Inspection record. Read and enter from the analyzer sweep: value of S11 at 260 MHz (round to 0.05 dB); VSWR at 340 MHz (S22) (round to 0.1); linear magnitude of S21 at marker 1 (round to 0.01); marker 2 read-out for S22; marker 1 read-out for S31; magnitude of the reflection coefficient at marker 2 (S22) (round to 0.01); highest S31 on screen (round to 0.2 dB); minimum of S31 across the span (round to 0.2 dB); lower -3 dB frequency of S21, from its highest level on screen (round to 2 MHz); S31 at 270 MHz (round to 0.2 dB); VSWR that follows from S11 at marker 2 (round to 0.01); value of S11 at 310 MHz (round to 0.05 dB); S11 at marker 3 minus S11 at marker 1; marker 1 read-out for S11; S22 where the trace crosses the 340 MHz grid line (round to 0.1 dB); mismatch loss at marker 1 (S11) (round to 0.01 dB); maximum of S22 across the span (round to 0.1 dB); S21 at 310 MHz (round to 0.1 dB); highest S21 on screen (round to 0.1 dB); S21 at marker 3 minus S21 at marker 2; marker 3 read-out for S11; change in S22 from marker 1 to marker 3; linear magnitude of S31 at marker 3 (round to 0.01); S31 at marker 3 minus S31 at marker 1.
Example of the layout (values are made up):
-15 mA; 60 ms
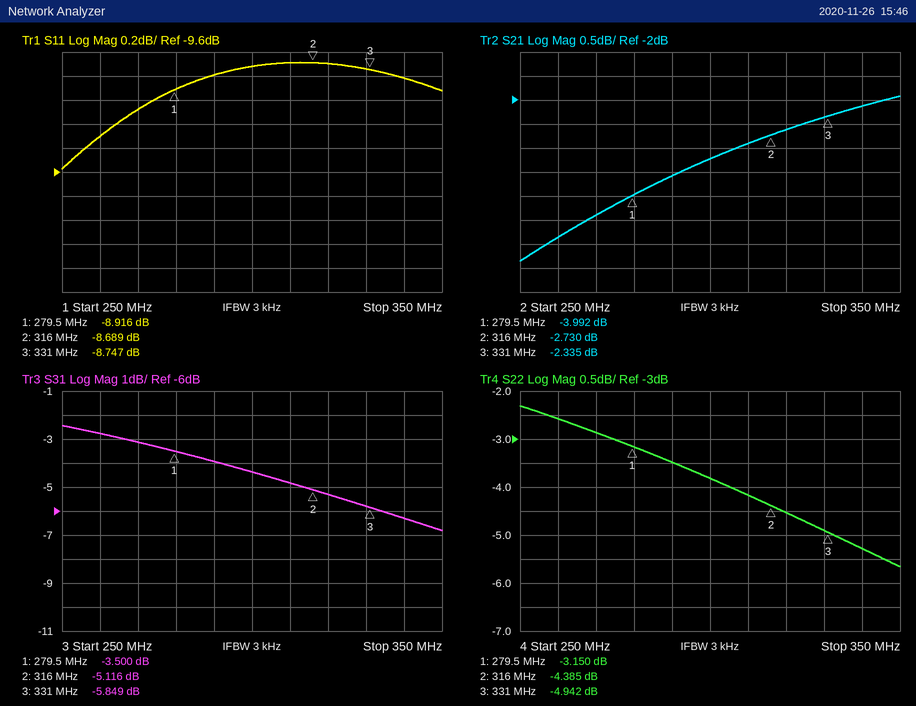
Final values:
-9.30 dB; 3.4; 0.63; -4.385 dB; -3.500 dB; 0.60; -2.4 dB; -6.8 dB; 258 MHz; -3.2 dB; 2.16; -8.70 dB; 0.169 dB; -8.916 dB; -5.3 dB; 0.60 dB; -2.3 dB; -2.9 dB; -1.9 dB; 0.395 dB; -8.747 dB; -1.792 dB; 0.51; -2.349 dB
